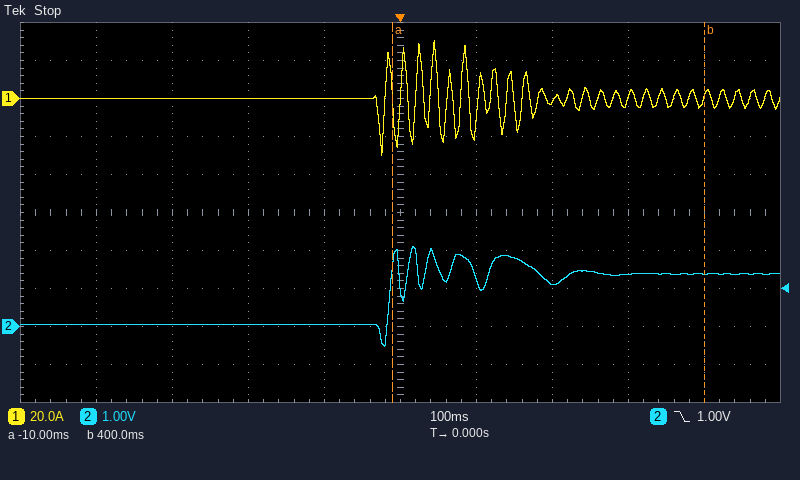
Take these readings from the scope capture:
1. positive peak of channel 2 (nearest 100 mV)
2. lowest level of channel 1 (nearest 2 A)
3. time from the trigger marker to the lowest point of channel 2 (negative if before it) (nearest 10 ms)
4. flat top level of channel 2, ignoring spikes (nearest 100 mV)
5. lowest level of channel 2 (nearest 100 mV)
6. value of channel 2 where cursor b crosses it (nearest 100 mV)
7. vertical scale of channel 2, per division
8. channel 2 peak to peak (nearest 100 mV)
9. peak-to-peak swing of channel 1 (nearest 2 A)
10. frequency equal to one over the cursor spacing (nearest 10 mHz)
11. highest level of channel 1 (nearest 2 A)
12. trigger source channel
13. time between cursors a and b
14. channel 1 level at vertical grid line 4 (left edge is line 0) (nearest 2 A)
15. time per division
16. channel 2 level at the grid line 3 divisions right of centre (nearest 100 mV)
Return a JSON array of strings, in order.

["2.1 V", "-30 A", "-20 ms", "1.4 V", "-500 mV", "1.4 V", "1 V", "2.6 V", "60 A", "2.44 Hz", "30 A", "channel 2", "410 ms", "0 A", "100 ms", "1.4 V"]
